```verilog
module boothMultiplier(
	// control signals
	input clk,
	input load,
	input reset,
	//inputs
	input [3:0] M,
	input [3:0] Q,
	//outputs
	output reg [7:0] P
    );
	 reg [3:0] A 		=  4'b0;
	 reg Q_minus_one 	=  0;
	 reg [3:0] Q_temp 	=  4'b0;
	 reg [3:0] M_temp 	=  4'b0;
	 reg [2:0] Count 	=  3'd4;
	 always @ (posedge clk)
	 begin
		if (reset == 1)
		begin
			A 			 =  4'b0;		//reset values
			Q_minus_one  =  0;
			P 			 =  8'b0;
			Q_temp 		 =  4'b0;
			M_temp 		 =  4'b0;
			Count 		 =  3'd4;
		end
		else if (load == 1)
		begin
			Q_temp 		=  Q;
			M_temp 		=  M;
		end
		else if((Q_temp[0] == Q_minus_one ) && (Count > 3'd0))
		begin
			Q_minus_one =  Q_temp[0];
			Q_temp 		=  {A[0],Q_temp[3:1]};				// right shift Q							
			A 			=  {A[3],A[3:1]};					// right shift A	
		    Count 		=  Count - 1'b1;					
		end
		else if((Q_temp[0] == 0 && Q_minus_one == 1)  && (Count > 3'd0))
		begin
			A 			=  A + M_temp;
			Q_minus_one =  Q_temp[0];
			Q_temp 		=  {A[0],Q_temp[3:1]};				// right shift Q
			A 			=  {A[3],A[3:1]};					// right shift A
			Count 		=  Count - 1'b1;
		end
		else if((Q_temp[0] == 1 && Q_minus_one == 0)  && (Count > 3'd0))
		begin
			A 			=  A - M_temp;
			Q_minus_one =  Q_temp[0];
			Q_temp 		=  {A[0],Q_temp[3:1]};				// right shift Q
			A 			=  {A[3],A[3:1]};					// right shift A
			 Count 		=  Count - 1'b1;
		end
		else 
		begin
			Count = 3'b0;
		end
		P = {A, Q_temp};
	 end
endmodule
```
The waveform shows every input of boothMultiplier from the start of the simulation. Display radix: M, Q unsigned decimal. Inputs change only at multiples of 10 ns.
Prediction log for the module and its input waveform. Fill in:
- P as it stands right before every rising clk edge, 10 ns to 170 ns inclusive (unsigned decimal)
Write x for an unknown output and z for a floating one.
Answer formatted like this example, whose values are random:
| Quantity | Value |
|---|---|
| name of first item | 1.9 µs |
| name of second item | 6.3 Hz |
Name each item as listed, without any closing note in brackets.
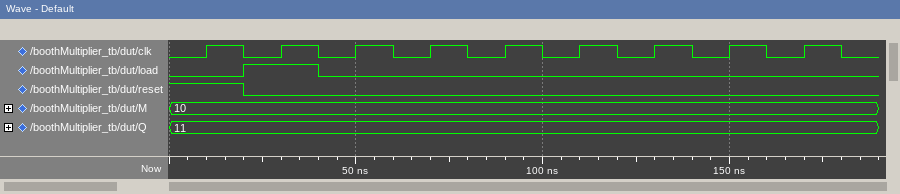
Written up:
| Quantity | Value |
|---|---|
| P as it stands right before every rising clk edge, 10 ns to 170 ns inclusive | x, 0, 11, 53, 26, 221, 30, 30, 30 |
